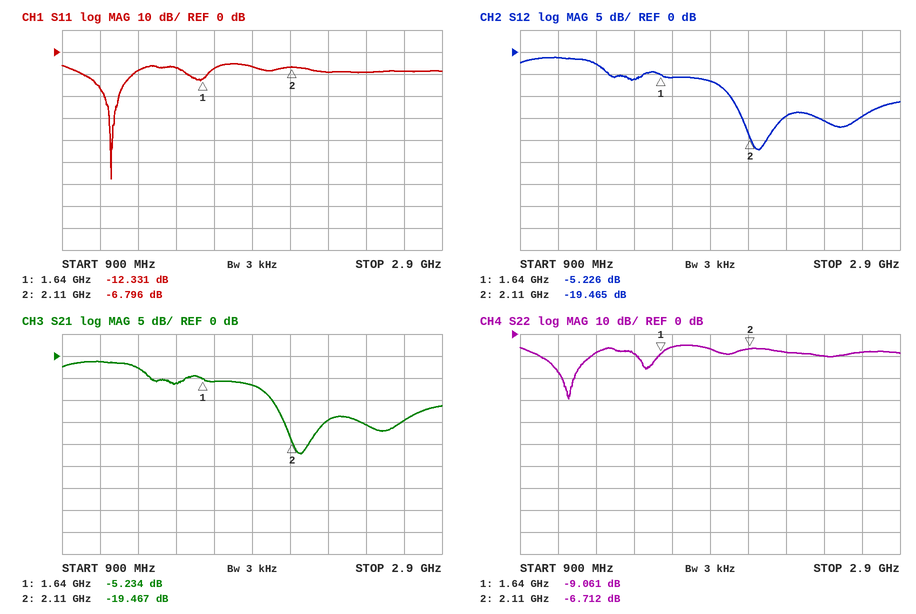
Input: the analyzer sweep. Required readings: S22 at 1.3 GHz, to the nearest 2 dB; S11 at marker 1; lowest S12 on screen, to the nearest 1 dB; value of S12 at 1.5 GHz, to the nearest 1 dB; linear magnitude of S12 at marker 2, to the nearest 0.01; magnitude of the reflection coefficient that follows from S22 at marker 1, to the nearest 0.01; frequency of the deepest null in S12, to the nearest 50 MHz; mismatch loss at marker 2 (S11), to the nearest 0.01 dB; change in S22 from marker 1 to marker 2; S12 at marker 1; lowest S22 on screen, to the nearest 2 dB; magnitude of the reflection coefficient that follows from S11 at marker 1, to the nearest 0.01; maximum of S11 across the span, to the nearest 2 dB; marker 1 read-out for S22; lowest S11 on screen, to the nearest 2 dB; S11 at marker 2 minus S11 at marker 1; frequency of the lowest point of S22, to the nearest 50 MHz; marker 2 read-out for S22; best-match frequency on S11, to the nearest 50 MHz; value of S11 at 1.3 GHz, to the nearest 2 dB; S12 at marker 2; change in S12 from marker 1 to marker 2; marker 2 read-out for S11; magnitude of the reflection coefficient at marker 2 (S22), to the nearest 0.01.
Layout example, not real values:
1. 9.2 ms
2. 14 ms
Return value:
1. -8 dB
2. -12.331 dB
3. -22 dB
4. -6 dB
5. 0.11
6. 0.35
7. 2.15 GHz
8. 1.02 dB
9. 2.349 dB
10. -5.226 dB
11. -30 dB
12. 0.24
13. -6 dB
14. -9.061 dB
15. -58 dB
16. 5.535 dB
17. 1.15 GHz
18. -6.712 dB
19. 1.15 GHz
20. -8 dB
21. -19.465 dB
22. -14.239 dB
23. -6.796 dB
24. 0.46
